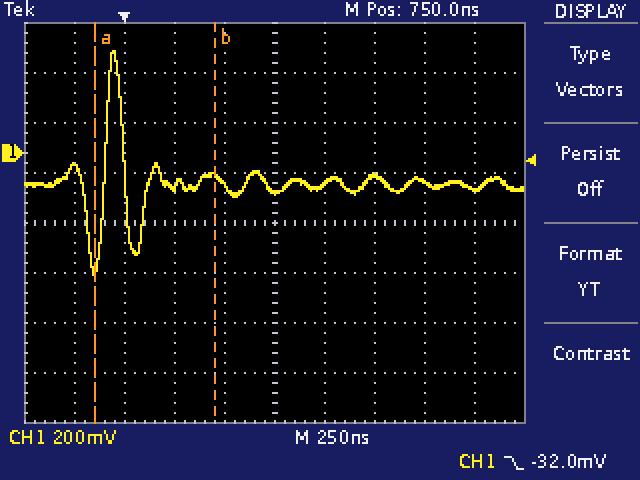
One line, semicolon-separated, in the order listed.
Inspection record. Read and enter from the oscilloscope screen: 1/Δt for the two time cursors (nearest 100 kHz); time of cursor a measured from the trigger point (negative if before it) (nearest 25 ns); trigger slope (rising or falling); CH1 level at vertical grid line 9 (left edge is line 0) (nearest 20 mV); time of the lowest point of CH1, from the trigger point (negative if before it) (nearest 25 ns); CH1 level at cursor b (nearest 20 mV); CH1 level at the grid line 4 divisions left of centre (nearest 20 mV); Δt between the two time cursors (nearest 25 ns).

1.7 MHz; -150 ns; falling; -140 mV; -150 ns; -100 mV; -60 mV; 600 ns
